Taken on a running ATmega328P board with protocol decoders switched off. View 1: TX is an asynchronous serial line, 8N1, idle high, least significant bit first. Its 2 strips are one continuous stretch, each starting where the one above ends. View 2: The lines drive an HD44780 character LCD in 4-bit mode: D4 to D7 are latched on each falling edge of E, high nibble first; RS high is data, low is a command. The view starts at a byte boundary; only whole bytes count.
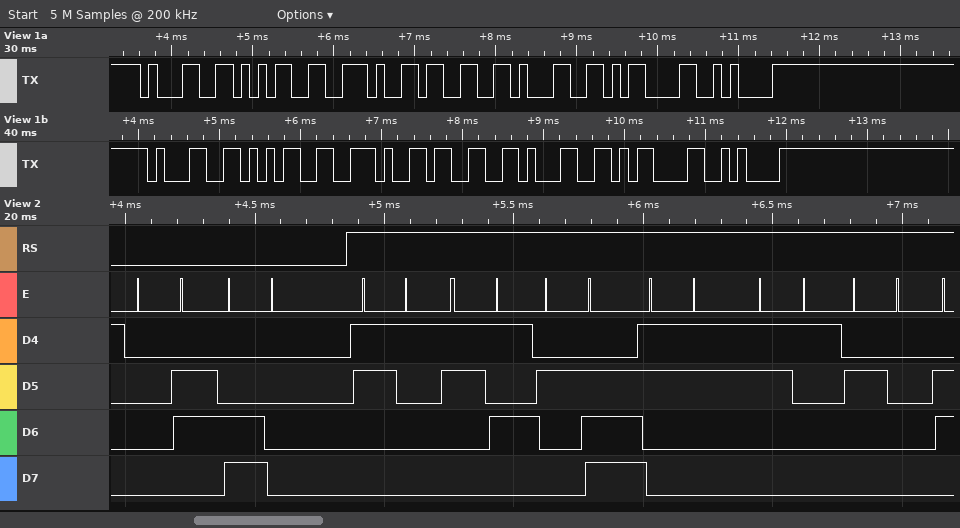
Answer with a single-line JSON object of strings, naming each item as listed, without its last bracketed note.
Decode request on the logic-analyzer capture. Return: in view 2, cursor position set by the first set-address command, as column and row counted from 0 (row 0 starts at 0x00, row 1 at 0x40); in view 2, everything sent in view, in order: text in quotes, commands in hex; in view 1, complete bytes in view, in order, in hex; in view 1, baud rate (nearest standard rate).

{"in view 2, cursor position set by the first set-address command, as column and row counted from 0": "column 0, row 1", "in view 2, everything sent in view, in order: text in quotes, commands in hex": "0x06 0xC0 \"15.31 \"", "in view 1, complete bytes in view, in order, in hex": "0x31 0x35 0x2E 0x33 0x31 0x0D 0x0A 0x31 0x35 0x2E 0x33 0x31 0x0D 0x0A", "in view 1, baud rate": "9600 baud"}
